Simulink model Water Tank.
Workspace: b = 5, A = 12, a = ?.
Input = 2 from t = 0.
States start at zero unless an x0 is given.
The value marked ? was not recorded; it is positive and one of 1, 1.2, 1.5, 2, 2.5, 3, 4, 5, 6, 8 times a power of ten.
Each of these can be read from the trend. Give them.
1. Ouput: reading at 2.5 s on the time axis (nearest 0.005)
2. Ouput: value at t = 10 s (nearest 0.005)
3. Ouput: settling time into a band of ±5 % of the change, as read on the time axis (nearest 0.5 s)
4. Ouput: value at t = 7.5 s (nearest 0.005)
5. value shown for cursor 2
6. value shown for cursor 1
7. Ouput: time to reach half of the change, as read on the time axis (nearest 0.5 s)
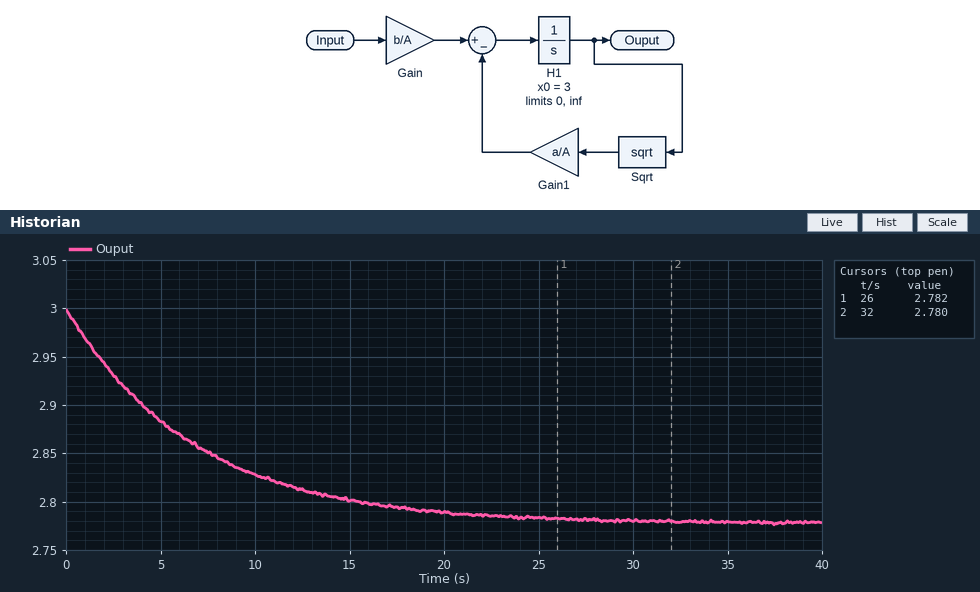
2.930
2.830
20.0 s
2.850
2.780
2.782
4.5 s
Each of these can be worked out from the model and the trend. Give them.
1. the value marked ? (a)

6
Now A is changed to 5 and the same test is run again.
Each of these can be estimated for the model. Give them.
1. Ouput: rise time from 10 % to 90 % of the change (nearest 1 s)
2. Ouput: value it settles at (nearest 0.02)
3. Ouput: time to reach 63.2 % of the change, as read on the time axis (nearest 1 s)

6 s
2.78
3 s
